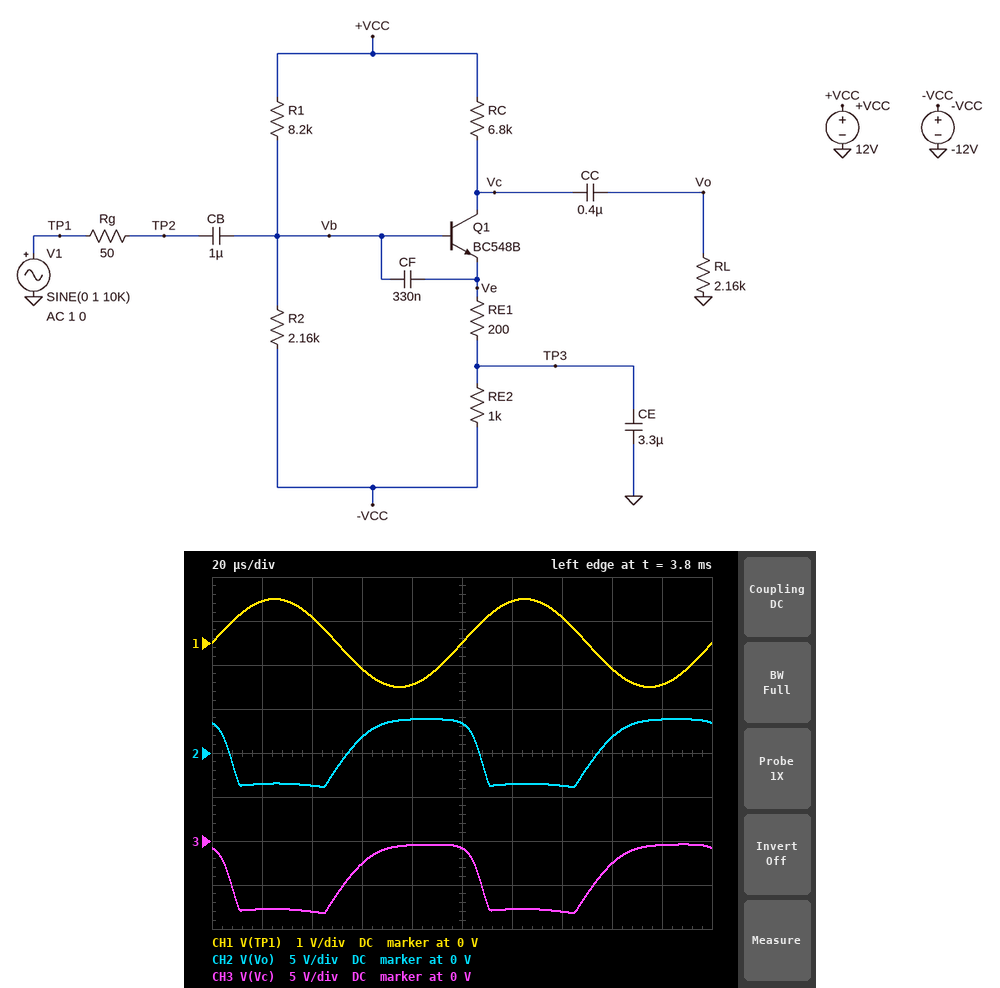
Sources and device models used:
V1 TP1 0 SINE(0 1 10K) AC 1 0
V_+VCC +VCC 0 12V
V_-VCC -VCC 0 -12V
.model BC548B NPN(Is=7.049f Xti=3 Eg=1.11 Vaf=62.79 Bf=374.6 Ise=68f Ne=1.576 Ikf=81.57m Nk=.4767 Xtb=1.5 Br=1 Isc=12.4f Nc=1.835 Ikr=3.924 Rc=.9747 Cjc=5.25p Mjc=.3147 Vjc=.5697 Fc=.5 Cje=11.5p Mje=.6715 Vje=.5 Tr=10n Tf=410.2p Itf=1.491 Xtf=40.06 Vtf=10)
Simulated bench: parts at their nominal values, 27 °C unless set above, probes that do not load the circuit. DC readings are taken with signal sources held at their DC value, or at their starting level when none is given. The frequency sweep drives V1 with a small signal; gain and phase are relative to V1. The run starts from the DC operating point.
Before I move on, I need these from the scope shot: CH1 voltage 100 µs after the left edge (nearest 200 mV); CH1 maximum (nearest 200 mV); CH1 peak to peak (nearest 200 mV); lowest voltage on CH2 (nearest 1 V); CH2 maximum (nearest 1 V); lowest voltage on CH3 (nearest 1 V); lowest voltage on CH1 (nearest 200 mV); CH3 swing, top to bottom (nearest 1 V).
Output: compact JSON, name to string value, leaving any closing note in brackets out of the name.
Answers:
{"CH1 voltage 100 µs after the left edge": "0 V", "CH1 maximum": "1.0 V", "CH1 peak to peak": "2.0 V", "lowest voltage on CH2": "-4 V", "CH2 maximum": "4 V", "lowest voltage on CH3": "-8 V", "lowest voltage on CH1": "-1.0 V", "CH3 swing, top to bottom": "8 V"}
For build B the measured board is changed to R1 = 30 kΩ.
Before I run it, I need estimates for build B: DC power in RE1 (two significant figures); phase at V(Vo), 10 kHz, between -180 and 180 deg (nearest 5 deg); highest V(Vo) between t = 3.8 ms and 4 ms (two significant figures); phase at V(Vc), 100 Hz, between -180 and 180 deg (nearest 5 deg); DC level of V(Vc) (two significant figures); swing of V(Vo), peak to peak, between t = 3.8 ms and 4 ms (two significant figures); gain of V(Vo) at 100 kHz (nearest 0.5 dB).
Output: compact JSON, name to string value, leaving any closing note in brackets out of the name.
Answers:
{"DC power in RE1": "130 µW", "phase at V(Vo), 10 kHz, between -180 and 180 deg": "145 deg", "highest V(Vo) between t = 3.8 ms and 4 ms": "1.4 V", "phase at V(Vc), 100 Hz, between -180 and 180 deg": "-140 deg", "DC level of V(Vc)": "6.6 V", "swing of V(Vo), peak to peak, between t = 3.8 ms and 4 ms": "6.7 V", "gain of V(Vo) at 100 kHz": "-0.5 dB"}
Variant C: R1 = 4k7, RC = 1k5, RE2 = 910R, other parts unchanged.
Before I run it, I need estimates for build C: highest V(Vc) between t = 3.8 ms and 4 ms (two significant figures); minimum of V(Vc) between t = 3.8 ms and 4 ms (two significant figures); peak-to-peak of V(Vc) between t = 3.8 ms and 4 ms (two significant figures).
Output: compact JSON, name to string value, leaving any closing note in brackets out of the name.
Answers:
{"highest V(Vc) between t = 3.8 ms and 4 ms": "6.7 V", "minimum of V(Vc) between t = 3.8 ms and 4 ms": "-1.3 V", "peak-to-peak of V(Vc) between t = 3.8 ms and 4 ms": "8.0 V"}
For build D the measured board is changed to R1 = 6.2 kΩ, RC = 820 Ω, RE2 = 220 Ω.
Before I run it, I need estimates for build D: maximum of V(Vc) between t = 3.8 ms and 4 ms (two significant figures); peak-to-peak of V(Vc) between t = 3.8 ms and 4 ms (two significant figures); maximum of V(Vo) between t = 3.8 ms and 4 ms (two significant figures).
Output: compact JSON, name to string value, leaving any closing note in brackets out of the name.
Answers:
{"maximum of V(Vc) between t = 3.8 ms and 4 ms": "4.3 V", "peak-to-peak of V(Vc) between t = 3.8 ms and 4 ms": "5.6 V", "maximum of V(Vo) between t = 3.8 ms and 4 ms": "2.8 V"}
